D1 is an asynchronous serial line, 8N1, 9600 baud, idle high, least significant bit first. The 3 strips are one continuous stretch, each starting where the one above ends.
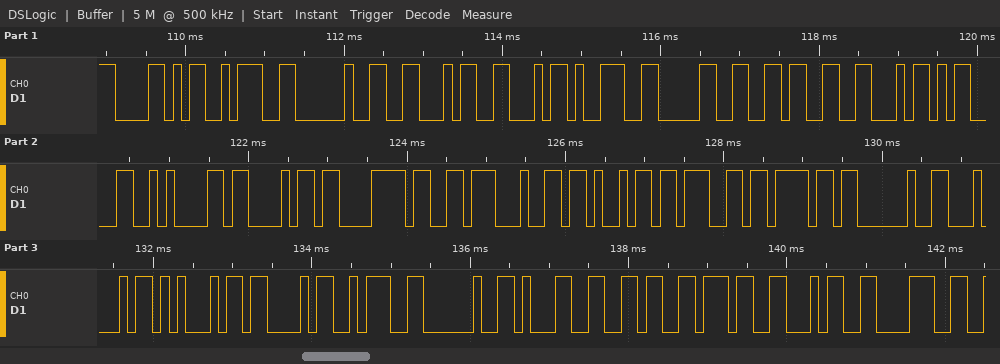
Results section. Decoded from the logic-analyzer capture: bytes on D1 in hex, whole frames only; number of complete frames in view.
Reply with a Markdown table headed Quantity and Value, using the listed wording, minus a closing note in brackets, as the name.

| Quantity | Value |
|---|---|
| bytes on D1 in hex, whole frames only | 58 3A 20 46 46 39 30 36 46 0D 0A 43 C3 B3 64 69 67 6F 20 44 45 43 3A 20 31 36 37 34 38 |
| number of complete frames in view | 29 |
